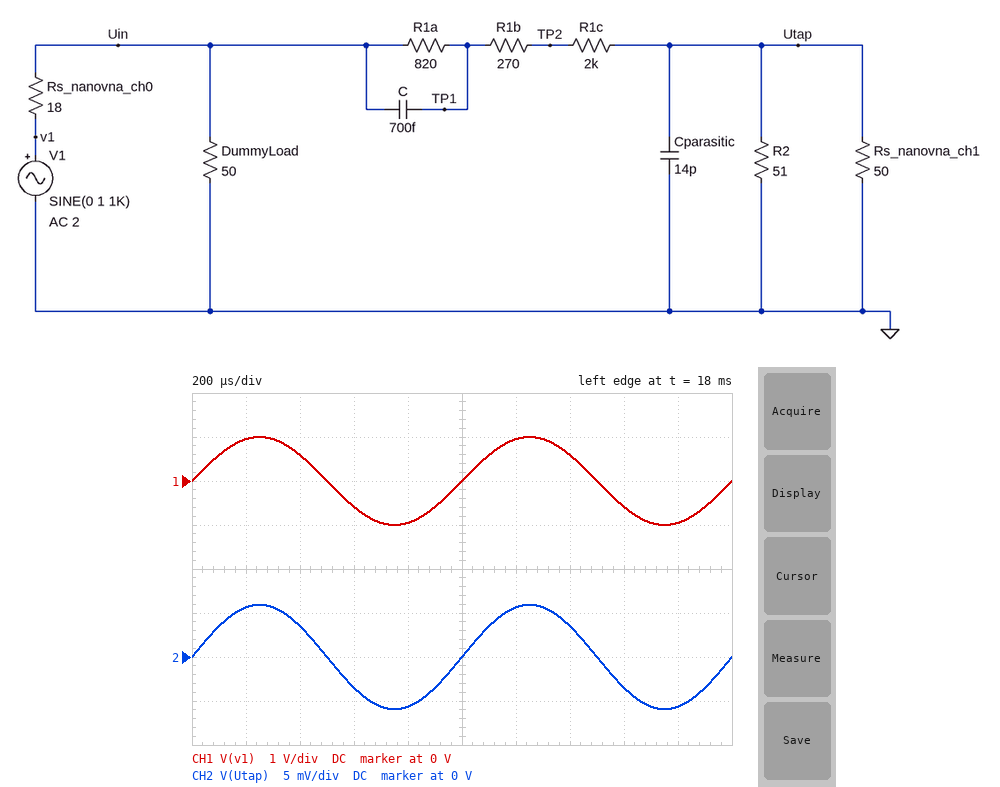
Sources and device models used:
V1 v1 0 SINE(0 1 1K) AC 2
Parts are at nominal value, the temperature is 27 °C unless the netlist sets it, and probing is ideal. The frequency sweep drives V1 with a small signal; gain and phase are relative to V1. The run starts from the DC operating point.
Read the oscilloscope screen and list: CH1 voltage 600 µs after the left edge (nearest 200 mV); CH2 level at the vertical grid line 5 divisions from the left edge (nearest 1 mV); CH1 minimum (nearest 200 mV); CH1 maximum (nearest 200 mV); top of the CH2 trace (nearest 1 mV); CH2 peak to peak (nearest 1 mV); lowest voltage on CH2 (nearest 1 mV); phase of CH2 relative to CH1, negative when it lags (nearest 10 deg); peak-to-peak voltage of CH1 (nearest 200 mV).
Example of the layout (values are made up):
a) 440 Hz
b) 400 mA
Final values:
a) -600 mV
b) 0 V
c) -1.0 V
d) 1.0 V
e) 6 mV
f) 12 mV
g) -6 mV
h) 0 deg
i) 2.0 V
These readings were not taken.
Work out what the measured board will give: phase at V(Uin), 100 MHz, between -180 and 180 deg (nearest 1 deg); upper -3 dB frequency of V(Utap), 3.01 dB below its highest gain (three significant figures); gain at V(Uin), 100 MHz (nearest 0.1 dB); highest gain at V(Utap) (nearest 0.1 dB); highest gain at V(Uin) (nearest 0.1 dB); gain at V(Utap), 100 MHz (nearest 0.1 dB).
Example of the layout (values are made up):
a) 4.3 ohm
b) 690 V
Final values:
a) 0 deg
b) 684 MHz
c) -2.7 dB
d) -44.5 dB
e) -2.7 dB
f) -44.5 dB
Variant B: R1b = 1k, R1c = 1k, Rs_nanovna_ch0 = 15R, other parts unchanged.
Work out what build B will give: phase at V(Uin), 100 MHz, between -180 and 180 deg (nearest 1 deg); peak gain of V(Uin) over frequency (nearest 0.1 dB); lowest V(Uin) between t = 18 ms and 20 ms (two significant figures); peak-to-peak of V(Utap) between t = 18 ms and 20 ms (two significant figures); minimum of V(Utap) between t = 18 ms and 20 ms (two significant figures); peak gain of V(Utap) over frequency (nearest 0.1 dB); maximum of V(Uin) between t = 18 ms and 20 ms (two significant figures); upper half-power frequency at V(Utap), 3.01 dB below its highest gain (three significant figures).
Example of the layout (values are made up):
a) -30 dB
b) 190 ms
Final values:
a) 0 deg
b) -2.3 dB
c) -770 mV
d) 14 mV
e) -6.8 mV
f) -43.3 dB
g) 770 mV
h) 711 MHz
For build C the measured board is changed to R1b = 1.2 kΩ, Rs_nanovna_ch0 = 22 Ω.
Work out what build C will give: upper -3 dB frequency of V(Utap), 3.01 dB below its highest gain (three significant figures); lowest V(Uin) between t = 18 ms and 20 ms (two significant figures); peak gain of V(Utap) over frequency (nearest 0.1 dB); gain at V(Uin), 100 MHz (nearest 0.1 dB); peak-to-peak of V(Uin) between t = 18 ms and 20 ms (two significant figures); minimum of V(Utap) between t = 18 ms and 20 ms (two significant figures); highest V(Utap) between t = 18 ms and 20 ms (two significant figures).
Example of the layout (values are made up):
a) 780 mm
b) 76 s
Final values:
a) 620 MHz
b) -690 mV
c) -47.3 dB
d) -3.2 dB
e) 1.4 V
f) -4.3 mV
g) 4.3 mV
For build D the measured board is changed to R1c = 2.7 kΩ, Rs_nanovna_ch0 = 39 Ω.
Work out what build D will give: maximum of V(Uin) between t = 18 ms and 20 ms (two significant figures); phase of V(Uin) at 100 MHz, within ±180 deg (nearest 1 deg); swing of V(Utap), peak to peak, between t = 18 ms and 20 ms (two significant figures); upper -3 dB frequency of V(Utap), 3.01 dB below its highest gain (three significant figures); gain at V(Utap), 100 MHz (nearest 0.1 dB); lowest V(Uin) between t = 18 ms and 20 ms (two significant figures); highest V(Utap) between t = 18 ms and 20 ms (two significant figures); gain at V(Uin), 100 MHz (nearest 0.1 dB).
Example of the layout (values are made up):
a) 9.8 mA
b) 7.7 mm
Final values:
a) 560 mV
b) 0 deg
c) 7.4 mV
d) 632 MHz
e) -48.7 dB
f) -560 mV
g) 3.7 mV
h) -5.1 dB
